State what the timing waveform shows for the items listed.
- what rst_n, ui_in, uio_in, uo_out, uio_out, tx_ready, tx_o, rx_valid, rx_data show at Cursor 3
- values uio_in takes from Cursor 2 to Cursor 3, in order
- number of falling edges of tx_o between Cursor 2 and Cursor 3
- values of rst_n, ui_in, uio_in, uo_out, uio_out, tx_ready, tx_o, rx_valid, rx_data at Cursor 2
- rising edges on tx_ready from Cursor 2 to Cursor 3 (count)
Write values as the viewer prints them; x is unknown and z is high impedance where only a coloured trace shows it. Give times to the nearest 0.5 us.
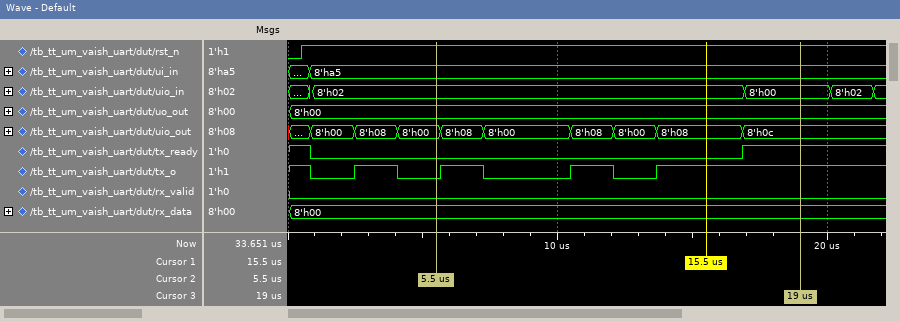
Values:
rst_n=1, ui_in=8'ha5, uio_in=8'h00, uo_out=8'h00, uio_out=8'h0c, tx_ready=1, tx_o=1, rx_valid=0, rx_data=8'h00
8'h02, 8'h00
2
rst_n=1, ui_in=8'ha5, uio_in=8'h02, uo_out=8'h00, uio_out=8'h00, tx_ready=0, tx_o=0, rx_valid=0, rx_data=8'h00
1
